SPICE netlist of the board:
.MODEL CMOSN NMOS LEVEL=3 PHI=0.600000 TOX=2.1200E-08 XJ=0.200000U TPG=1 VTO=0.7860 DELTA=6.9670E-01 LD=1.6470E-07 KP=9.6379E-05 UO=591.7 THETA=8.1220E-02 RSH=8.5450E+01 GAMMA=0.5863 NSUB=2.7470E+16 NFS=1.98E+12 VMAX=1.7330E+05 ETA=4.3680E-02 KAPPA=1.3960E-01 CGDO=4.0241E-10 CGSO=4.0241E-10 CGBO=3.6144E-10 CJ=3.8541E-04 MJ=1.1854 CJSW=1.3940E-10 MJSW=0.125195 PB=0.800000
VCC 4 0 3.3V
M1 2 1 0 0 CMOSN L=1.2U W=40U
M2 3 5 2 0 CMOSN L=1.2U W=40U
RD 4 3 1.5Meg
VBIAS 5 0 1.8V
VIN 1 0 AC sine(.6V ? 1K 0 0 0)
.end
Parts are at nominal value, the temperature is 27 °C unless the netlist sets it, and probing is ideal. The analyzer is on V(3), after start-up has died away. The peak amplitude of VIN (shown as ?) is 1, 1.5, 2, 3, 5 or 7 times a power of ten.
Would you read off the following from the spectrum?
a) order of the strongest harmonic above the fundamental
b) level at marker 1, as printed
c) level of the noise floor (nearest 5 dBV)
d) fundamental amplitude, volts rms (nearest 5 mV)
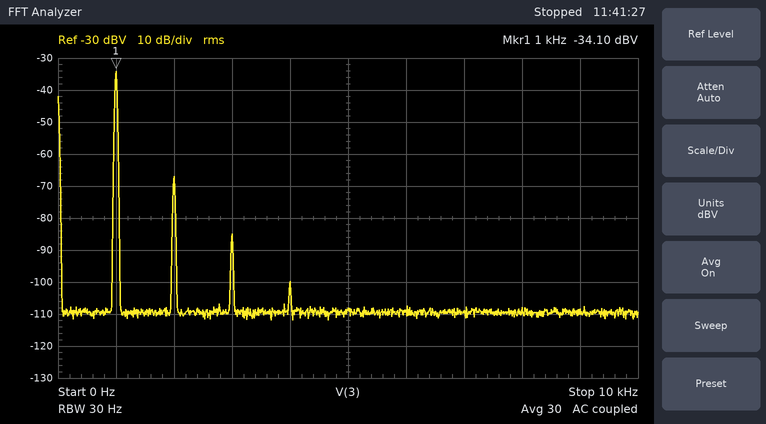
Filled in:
2
-34.10 dBV
-110 dBV
20 mV
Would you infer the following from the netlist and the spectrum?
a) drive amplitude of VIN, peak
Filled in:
1.5 mV
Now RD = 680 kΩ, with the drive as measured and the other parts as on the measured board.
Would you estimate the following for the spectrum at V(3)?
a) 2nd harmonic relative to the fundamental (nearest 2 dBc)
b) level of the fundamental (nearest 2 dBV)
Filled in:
-48 dBc
-38 dBV
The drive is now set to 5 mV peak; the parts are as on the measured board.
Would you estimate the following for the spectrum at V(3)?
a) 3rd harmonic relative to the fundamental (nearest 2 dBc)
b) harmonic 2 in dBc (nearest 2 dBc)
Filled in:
-38 dBc
-22 dBc
